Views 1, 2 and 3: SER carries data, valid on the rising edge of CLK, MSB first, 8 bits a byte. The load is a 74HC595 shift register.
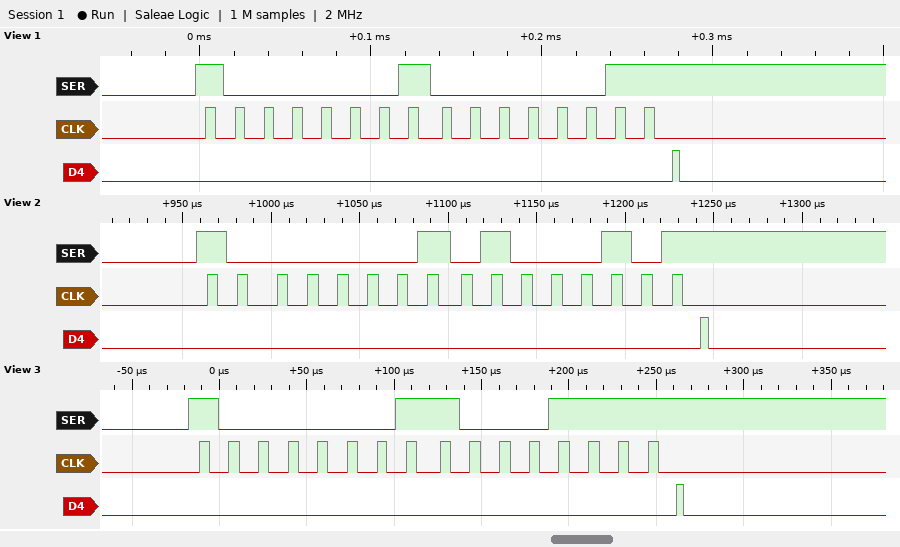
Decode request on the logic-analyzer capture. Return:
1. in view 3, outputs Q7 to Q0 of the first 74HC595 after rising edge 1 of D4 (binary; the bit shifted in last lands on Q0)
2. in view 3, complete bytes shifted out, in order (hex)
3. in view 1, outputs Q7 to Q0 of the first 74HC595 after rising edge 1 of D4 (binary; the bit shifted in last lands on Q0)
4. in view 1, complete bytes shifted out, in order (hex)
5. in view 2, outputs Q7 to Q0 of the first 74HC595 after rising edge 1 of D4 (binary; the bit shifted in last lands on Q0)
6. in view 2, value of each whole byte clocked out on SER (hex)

10001111
81 8F
00000011
81 03
01000101
81 45
